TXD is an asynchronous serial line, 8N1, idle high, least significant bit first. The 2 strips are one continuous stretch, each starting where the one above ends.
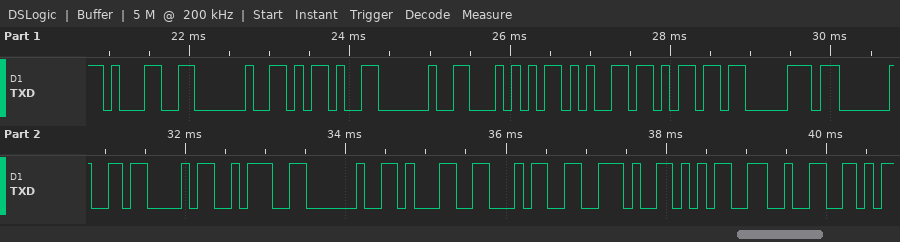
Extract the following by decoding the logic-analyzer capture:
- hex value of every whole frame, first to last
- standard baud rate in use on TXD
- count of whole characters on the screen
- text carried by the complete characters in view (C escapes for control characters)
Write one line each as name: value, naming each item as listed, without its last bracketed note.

hex value of every whole frame, first to last: 31 20 2D 20 54 65 6D 70 20 43 3A 20 31 34 2E 35 32
standard baud rate in use on TXD: 9600 baud
count of whole characters on the screen: 17
text carried by the complete characters in view: "1 - Temp C: 14.52"
